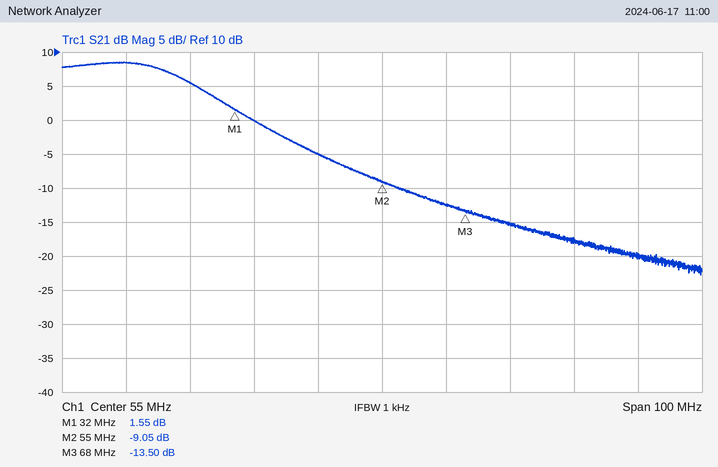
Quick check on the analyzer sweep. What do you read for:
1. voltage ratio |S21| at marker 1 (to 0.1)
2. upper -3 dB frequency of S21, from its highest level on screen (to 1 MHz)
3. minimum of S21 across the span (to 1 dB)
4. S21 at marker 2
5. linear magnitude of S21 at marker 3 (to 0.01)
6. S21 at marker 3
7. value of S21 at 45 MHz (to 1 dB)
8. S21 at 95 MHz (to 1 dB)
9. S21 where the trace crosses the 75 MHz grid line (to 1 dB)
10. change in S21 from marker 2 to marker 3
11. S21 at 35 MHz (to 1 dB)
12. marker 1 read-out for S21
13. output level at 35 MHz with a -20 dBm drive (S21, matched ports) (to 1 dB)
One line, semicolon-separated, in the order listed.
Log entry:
1.2; 25 MHz; -23 dB; -9.05 dB; 0.21; -13.50 dB; -5 dB; -20 dB; -15 dB; -4.45 dB; 0 dB; 1.55 dB; -20 dBm
